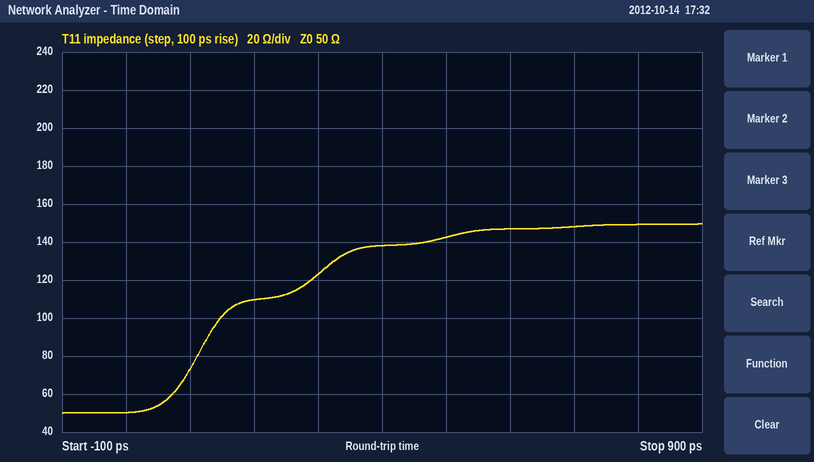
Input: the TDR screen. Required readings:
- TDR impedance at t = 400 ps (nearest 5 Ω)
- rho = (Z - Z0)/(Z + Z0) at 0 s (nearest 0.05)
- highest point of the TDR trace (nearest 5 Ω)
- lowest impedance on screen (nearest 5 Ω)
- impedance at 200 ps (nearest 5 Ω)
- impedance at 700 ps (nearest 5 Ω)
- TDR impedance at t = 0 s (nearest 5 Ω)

140 Ω
0.00
150 Ω
50 Ω
110 Ω
150 Ω
50 Ω
